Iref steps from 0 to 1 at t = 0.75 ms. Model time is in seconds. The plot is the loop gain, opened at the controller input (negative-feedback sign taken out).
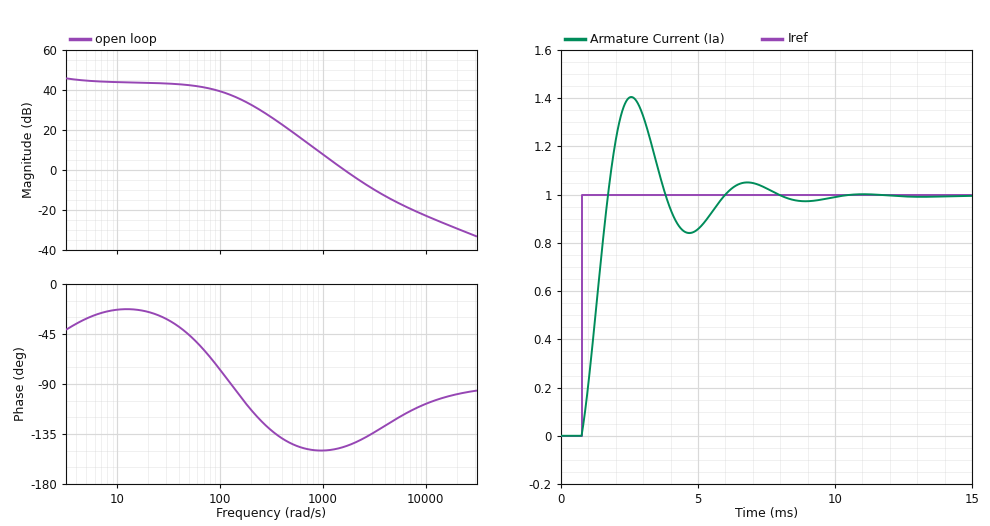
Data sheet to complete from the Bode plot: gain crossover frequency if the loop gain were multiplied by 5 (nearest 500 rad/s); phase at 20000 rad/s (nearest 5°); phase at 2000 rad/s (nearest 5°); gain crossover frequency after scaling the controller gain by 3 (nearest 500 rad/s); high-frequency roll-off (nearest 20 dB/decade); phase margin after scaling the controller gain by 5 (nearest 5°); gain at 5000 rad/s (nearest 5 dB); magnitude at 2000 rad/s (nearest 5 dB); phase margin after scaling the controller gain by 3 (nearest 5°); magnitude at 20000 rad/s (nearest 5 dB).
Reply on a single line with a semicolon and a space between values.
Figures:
4500 rad/s; -100°; -145°; 3000 rad/s; -20 dB/decade; 55°; -15 dB; -5 dB; 45°; -30 dB
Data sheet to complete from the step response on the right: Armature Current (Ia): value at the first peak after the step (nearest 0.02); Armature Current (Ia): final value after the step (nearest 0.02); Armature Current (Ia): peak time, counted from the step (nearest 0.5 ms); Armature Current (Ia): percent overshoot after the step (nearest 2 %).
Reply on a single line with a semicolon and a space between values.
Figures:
1.40; 1.00; 2.0 ms; 42 %
